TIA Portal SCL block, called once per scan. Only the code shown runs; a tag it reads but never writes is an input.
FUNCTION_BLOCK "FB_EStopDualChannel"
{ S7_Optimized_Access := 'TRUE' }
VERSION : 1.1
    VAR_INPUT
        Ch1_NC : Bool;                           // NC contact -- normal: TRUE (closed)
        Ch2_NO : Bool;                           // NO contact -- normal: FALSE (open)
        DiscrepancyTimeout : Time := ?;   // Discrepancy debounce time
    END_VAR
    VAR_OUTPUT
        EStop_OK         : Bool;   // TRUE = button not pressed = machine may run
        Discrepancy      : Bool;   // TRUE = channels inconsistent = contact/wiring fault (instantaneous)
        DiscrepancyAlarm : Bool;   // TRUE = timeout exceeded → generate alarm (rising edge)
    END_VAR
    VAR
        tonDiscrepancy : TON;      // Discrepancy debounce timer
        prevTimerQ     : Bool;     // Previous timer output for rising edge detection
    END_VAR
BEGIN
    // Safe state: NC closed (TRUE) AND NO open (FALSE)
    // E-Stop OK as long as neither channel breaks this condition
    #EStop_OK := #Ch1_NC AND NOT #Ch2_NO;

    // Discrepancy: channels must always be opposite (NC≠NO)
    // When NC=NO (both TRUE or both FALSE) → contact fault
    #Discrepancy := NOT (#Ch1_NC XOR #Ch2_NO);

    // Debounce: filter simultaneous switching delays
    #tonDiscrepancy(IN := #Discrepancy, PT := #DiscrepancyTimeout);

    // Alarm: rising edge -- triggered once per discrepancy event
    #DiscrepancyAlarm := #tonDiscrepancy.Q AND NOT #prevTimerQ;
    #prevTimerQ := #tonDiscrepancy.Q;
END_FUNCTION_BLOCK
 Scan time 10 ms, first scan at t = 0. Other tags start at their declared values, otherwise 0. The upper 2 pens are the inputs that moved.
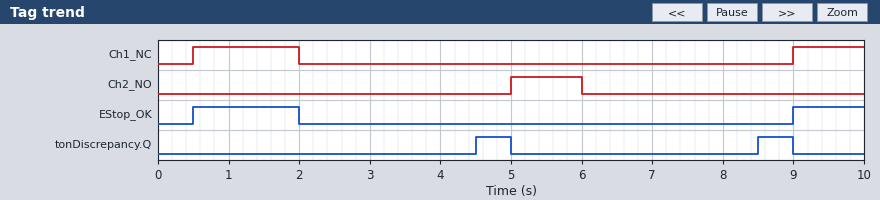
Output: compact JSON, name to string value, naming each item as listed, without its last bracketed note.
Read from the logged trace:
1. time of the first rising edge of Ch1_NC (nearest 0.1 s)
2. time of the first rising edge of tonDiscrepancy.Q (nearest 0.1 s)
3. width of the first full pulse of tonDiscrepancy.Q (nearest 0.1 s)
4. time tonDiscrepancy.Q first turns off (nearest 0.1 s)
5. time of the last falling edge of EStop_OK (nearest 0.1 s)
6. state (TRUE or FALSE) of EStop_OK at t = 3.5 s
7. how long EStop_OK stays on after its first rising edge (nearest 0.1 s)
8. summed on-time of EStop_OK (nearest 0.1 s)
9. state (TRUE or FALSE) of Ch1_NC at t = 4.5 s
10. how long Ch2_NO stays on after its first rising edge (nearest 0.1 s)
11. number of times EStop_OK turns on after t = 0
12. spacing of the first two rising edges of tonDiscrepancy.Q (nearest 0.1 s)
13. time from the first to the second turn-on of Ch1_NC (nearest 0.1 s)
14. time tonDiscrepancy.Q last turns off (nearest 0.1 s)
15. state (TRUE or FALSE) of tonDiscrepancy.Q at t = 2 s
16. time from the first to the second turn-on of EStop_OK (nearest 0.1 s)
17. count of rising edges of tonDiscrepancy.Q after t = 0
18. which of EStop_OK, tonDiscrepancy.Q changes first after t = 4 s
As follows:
{"time of the first rising edge of Ch1_NC": "0.5 s", "time of the first rising edge of tonDiscrepancy.Q": "4.5 s", "width of the first full pulse of tonDiscrepancy.Q": "0.5 s", "time tonDiscrepancy.Q first turns off": "5.0 s", "time of the last falling edge of EStop_OK": "2.0 s", "state (TRUE or FALSE) of EStop_OK at t = 3.5 s": "FALSE", "how long EStop_OK stays on after its first rising edge": "1.5 s", "summed on-time of EStop_OK": "2.5 s", "state (TRUE or FALSE) of Ch1_NC at t = 4.5 s": "FALSE", "how long Ch2_NO stays on after its first rising edge": "1.0 s", "number of times EStop_OK turns on after t = 0": "2", "spacing of the first two rising edges of tonDiscrepancy.Q": "4.0 s", "time from the first to the second turn-on of Ch1_NC": "8.5 s", "time tonDiscrepancy.Q last turns off": "9.0 s", "state (TRUE or FALSE) of tonDiscrepancy.Q at t = 2 s": "FALSE", "time from the first to the second turn-on of EStop_OK": "8.5 s", "count of rising edges of tonDiscrepancy.Q after t = 0": "2", "which of EStop_OK, tonDiscrepancy.Q changes first after t = 4 s": "tonDiscrepancy.Q"}
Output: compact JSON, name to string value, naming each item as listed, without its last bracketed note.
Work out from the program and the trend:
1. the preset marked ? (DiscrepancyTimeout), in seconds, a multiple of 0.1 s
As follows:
{"the preset marked ? (DiscrepancyTimeout), in seconds, a multiple of 0.1 s": "2.5 s"}
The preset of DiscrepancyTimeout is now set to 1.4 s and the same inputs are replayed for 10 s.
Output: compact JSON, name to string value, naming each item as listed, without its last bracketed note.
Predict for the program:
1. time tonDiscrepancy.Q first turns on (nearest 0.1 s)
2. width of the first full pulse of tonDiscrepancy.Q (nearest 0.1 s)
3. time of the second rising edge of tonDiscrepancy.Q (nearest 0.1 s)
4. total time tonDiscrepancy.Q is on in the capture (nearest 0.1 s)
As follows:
{"time tonDiscrepancy.Q first turns on": "3.4 s", "width of the first full pulse of tonDiscrepancy.Q": "1.6 s", "time of the second rising edge of tonDiscrepancy.Q": "7.4 s", "total time tonDiscrepancy.Q is on in the capture": "3.2 s"}
